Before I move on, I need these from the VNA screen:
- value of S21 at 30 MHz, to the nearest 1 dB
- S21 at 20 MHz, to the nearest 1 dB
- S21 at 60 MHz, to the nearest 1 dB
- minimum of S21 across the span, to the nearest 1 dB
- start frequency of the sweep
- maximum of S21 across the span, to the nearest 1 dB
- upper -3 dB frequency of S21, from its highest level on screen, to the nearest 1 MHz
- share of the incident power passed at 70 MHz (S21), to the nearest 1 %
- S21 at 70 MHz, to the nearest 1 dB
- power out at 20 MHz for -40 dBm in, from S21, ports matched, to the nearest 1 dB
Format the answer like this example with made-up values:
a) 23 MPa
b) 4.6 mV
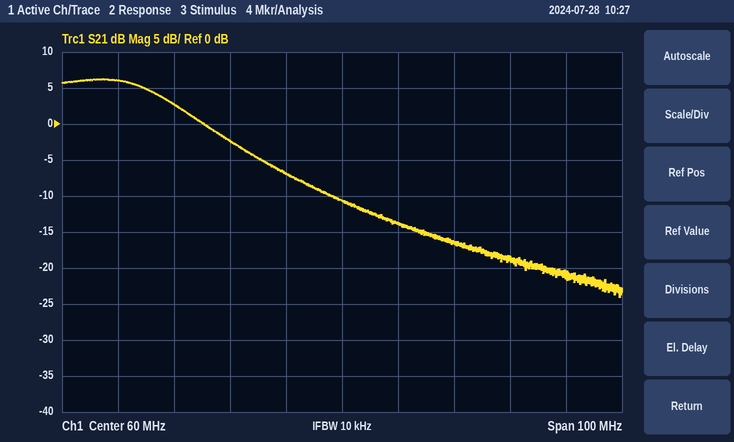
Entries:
a) 3 dB
b) 6 dB
c) -11 dB
d) -24 dB
e) 10 MHz
f) 6 dB
g) 29 MHz
h) 4 %
i) -14 dB
j) -34 dBm
